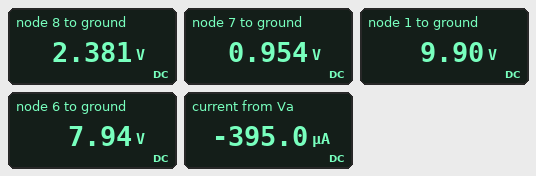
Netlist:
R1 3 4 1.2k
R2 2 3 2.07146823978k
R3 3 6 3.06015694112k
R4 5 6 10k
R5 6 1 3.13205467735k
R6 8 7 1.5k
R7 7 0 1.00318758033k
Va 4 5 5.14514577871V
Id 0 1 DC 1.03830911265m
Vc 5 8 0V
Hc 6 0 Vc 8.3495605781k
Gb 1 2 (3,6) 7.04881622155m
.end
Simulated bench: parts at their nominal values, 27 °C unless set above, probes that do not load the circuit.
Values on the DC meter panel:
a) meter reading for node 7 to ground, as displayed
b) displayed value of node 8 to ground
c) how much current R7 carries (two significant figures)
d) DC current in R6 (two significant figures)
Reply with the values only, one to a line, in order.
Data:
0.954 V
2.381 V
950 µA
950 µA
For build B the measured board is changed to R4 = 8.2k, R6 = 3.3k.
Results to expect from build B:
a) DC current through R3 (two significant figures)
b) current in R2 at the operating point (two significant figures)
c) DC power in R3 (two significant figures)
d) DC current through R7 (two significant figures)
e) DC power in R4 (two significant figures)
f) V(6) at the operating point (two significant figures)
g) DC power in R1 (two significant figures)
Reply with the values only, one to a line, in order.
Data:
36 µA
780 µA
4.0 µW
1.5 mA
4.3 mW
12 V
660 µW
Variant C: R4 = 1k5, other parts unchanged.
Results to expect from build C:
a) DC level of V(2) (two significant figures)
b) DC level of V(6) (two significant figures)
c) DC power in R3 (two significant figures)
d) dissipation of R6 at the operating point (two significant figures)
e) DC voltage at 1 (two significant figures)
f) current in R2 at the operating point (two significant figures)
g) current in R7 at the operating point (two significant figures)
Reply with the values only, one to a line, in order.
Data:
940 mV
4.8 V
20 µW
500 µW
14 V
1.8 mA
580 µA
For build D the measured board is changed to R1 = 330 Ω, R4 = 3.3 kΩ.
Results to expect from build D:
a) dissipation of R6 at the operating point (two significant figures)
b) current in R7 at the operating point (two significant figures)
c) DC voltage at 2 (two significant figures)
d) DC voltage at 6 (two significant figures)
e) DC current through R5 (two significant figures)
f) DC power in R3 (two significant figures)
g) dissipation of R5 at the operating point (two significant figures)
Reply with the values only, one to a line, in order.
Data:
1.1 mW
860 µA
5.6 V
7.2 V
1.7 mA
3.2 µW
9.4 mW
